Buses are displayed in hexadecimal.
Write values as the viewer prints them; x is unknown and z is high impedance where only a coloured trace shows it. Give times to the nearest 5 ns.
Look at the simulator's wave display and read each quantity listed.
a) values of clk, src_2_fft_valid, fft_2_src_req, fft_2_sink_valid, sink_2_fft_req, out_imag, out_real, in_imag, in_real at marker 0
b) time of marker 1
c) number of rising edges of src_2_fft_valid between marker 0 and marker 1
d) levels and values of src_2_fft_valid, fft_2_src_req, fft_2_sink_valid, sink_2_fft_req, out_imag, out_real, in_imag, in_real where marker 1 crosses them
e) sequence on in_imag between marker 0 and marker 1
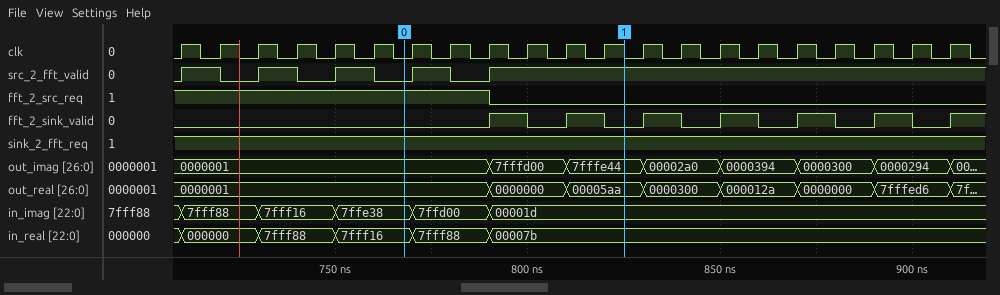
clk=0, src_2_fft_valid=0, fft_2_src_req=1, fft_2_sink_valid=0, sink_2_fft_req=1, out_imag=0000001, out_real=0000001, in_imag=7ffe38, in_real=7fff16
825 ns
2
src_2_fft_valid=1, fft_2_src_req=0, fft_2_sink_valid=0, sink_2_fft_req=1, out_imag=7fffe44, out_real=00005aa, in_imag=00001d, in_real=00007b
7ffe38, 7ffd00, 00001d
